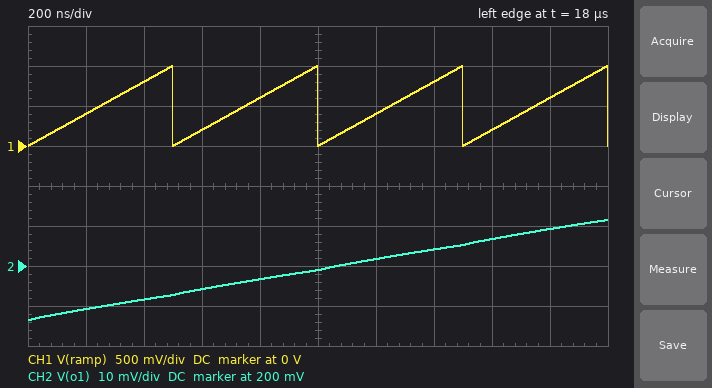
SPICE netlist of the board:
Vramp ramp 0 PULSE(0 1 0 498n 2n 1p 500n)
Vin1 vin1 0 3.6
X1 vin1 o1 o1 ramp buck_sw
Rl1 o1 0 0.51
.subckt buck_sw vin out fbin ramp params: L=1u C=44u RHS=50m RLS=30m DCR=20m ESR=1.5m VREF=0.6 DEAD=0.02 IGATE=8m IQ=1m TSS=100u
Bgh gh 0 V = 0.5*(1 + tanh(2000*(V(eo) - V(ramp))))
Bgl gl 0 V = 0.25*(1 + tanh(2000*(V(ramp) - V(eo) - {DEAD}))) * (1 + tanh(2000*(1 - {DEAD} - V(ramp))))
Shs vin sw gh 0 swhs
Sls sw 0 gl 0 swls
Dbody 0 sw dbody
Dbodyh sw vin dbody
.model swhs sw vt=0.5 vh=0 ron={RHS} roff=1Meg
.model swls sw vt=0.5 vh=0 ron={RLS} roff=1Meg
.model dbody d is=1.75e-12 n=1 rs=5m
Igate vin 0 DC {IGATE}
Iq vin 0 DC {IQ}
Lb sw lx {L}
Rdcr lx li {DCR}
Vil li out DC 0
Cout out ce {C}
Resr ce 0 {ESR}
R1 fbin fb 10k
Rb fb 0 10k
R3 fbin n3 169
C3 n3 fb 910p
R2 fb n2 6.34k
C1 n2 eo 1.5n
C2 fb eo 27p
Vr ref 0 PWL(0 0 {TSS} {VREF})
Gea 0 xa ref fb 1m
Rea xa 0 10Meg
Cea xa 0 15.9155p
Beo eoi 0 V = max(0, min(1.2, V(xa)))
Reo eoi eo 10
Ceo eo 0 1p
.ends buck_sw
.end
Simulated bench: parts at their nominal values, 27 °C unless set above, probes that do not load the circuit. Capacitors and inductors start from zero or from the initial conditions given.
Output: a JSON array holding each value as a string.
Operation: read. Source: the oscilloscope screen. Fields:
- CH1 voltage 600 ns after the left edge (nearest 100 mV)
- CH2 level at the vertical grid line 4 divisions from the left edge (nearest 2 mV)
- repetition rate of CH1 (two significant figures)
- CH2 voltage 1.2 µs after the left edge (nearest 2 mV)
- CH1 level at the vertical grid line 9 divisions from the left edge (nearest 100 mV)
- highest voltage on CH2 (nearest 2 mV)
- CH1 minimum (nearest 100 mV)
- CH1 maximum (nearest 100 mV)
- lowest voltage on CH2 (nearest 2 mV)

["200 mV", "196 mV", "2.0 MHz", "202 mV", "600 mV", "212 mV", "0 V", "1.0 V", "186 mV"]
